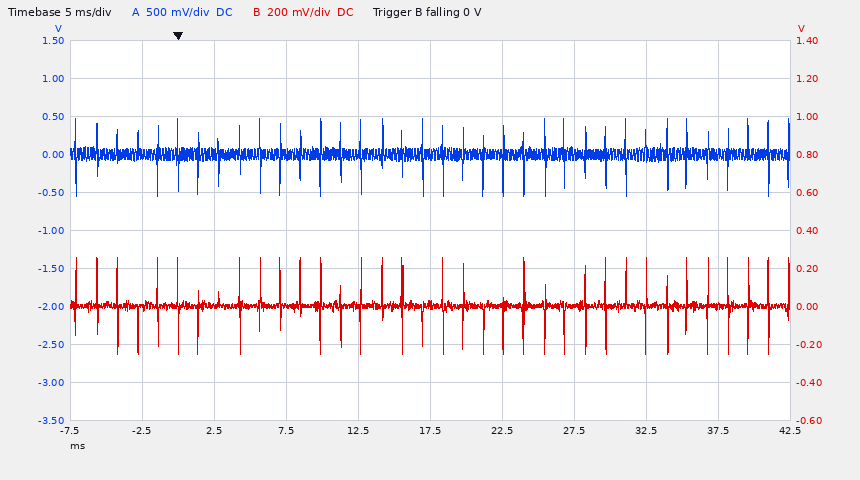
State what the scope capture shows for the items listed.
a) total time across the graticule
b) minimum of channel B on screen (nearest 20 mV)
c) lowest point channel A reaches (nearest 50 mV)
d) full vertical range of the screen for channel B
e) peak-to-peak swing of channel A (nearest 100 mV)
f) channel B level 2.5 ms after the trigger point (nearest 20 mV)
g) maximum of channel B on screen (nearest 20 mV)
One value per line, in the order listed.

50 ms
-260 mV
-550 mV
2 V
1.00 V
0 mV
260 mV
